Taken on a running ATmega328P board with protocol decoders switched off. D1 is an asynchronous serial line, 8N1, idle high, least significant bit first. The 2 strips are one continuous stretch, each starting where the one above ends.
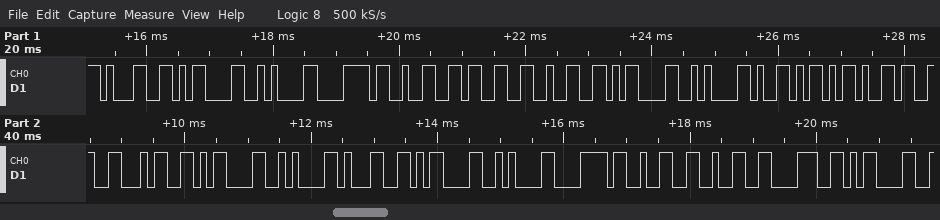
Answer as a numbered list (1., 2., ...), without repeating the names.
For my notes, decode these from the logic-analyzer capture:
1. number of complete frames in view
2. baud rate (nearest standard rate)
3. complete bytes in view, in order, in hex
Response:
1. 23
2. 9600 baud
3. 31 0D 0A 78 32 33 32 0D 0A 59 2D 33 34 0D 0A 31 0D 0A 78 32 32 38 0D
